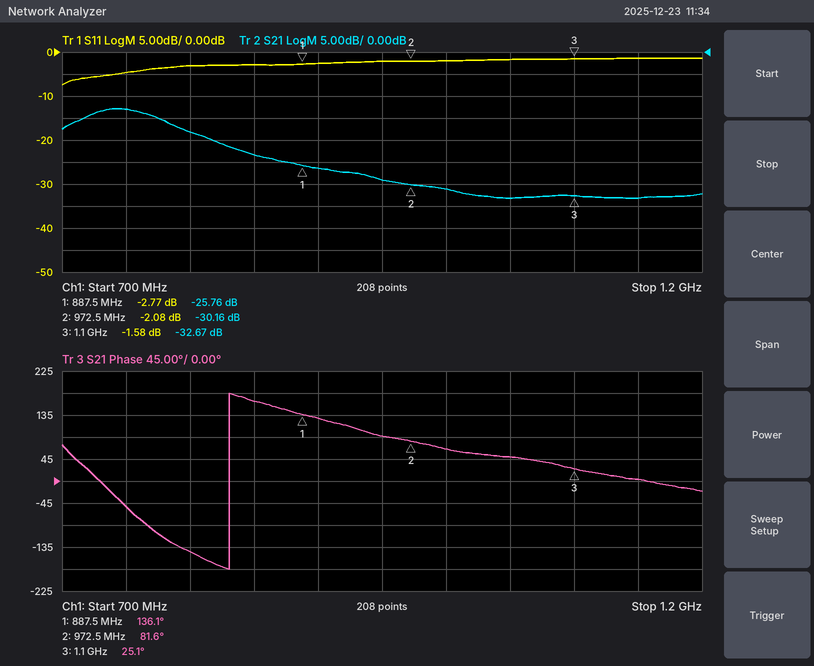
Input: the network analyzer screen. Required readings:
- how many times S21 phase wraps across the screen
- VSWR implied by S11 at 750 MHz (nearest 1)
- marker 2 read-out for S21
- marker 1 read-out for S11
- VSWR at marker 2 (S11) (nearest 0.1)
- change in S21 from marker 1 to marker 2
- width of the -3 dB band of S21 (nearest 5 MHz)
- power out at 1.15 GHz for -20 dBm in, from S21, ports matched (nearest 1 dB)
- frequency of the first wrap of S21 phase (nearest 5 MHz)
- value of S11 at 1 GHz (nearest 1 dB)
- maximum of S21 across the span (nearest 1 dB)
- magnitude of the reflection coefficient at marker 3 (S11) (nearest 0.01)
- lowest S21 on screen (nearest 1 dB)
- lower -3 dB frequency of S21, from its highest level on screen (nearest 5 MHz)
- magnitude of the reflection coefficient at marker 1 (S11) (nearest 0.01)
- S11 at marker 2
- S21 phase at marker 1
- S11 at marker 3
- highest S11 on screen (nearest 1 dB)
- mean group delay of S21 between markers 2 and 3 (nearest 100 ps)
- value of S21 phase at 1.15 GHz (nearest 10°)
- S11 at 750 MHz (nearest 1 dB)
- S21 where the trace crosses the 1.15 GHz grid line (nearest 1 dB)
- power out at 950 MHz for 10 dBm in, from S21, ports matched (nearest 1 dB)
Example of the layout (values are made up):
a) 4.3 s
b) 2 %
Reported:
a) 1
b) 4
c) -30.16 dB
d) -2.77 dB
e) 8.4
f) -4.40 dB
g) 70 MHz
h) -53 dBm
i) 830 MHz
j) -2 dB
k) -13 dB
l) 0.83
m) -33 dB
n) 710 MHz
o) 0.73
p) -2.08 dB
q) 136.1°
r) -1.58 dB
s) -1 dB
t) 1.2 ns
u) 0°
v) -5 dB
w) -33 dB
x) -19 dBm
